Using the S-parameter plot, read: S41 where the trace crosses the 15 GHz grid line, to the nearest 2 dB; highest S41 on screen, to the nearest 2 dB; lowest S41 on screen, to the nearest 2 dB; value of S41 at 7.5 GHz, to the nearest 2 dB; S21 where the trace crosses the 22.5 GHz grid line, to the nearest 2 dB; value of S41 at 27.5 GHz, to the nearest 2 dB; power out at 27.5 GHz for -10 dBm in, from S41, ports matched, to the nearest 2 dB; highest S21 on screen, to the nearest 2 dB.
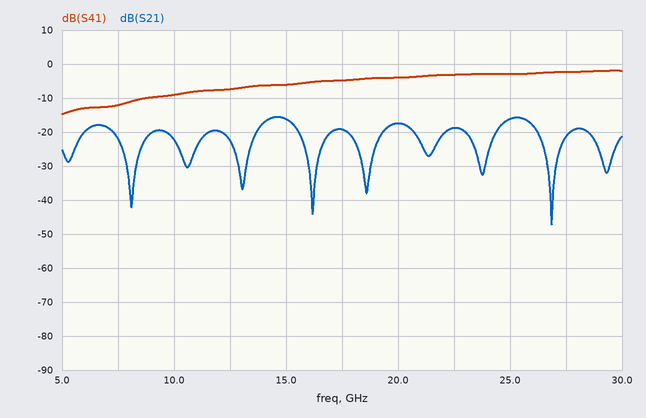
-6 dB
-2 dB
-14 dB
-12 dB
-18 dB
-2 dB
-12 dBm
-16 dB
